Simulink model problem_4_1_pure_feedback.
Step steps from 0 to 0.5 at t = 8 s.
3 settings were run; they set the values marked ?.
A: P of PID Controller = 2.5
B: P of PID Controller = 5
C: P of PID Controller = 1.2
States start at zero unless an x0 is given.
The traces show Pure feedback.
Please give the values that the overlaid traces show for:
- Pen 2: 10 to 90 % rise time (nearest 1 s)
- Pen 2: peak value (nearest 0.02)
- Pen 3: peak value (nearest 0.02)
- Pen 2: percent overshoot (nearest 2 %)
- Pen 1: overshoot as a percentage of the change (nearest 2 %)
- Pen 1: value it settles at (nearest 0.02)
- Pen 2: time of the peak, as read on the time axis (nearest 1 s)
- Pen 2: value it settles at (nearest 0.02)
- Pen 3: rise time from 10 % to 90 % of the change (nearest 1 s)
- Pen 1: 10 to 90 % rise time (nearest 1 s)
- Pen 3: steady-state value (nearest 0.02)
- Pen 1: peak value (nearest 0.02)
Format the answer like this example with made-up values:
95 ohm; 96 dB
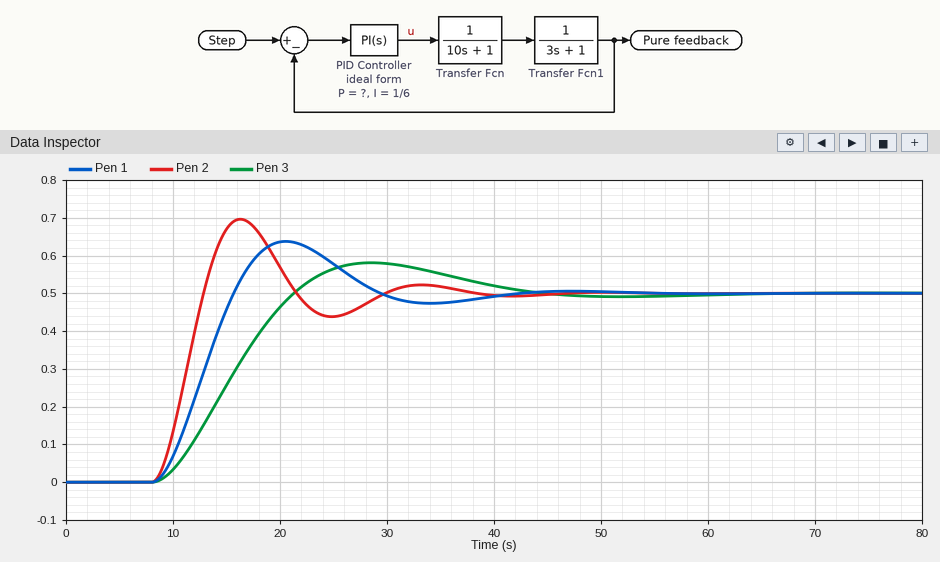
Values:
3 s; 0.70; 0.58; 40 %; 28 %; 0.50; 16 s; 0.50; 9 s; 5 s; 0.50; 0.64
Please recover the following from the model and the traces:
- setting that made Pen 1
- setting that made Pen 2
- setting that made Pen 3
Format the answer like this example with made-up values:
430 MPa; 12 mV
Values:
A; B; C
